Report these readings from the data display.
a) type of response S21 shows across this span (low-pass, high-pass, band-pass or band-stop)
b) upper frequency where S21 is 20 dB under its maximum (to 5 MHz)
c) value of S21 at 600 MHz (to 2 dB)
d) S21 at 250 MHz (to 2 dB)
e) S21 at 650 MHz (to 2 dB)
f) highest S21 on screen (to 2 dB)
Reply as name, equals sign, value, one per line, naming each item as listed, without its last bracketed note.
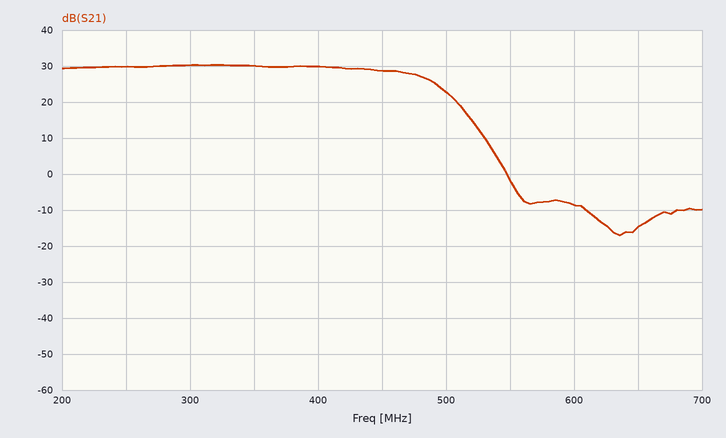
type of response S21 shows across this span = low-pass
upper frequency where S21 is 20 dB under its maximum = 530 MHz
value of S21 at 600 MHz = -8 dB
S21 at 250 MHz = 30 dB
S21 at 650 MHz = -14 dB
highest S21 on screen = 30 dB
